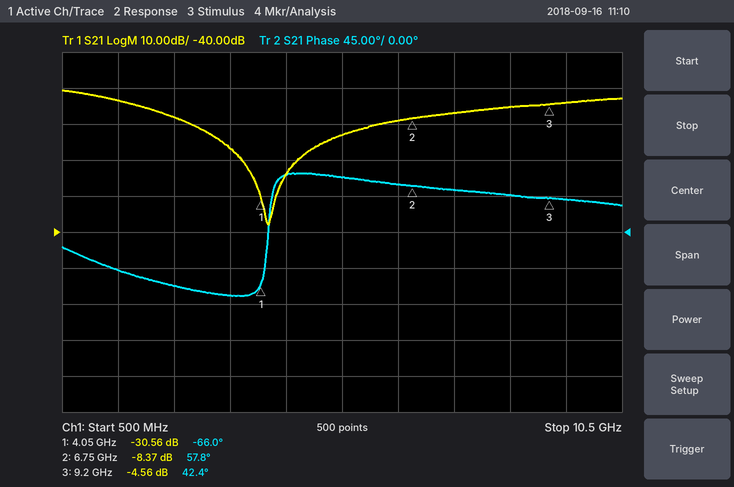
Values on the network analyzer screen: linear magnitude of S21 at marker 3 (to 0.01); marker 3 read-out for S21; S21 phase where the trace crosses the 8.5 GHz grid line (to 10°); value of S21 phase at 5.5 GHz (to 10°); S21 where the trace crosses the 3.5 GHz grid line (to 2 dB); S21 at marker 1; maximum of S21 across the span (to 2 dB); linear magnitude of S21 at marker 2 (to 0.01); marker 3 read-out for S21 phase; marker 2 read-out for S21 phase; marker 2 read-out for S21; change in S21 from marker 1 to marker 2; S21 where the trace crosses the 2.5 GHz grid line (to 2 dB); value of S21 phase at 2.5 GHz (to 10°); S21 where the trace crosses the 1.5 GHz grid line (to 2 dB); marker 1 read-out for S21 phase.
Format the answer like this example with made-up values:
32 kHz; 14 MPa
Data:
0.59; -4.56 dB; 50°; 70°; -16 dB; -30.56 dB; 0 dB; 0.38; 42.4°; 57.8°; -8.37 dB; 22.19 dB; -8 dB; -70°; -4 dB; -66.0°
